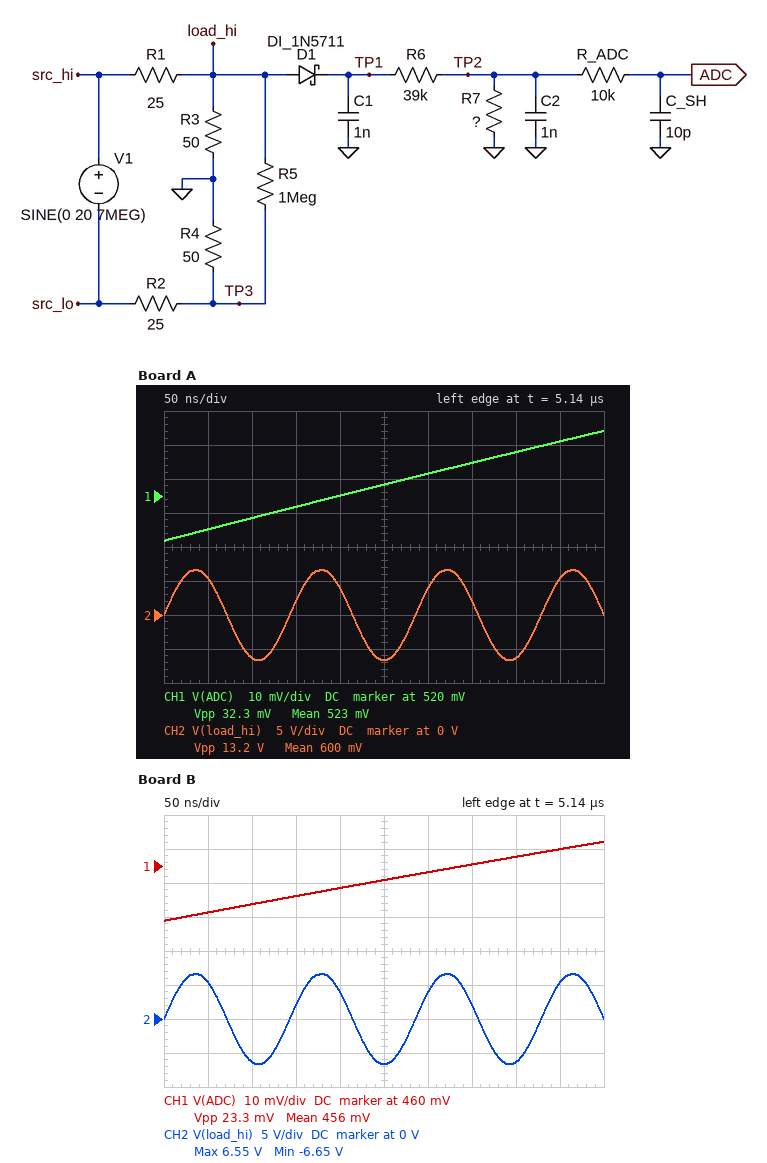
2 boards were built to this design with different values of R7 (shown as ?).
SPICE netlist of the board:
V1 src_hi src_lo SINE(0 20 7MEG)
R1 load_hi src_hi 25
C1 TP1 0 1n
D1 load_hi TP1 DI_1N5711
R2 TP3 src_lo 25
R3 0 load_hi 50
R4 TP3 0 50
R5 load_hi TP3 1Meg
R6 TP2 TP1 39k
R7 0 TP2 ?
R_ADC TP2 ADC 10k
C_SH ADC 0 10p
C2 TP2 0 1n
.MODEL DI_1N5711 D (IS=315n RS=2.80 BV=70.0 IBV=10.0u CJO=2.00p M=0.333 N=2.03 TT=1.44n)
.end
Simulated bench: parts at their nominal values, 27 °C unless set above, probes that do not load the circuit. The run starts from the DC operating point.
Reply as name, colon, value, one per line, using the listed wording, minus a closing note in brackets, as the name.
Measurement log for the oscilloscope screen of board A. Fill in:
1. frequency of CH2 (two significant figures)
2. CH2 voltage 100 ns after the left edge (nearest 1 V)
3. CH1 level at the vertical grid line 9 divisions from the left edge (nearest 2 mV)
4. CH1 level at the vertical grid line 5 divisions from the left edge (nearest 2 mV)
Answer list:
frequency of CH2: 7.0 MHz
CH2 voltage 100 ns after the left edge: -6 V
CH1 level at the vertical grid line 9 divisions from the left edge: 536 mV
CH1 level at the vertical grid line 5 divisions from the left edge: 524 mV
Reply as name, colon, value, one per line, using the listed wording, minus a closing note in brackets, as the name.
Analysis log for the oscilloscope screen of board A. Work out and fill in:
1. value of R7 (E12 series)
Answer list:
value of R7: 6.8 kΩ
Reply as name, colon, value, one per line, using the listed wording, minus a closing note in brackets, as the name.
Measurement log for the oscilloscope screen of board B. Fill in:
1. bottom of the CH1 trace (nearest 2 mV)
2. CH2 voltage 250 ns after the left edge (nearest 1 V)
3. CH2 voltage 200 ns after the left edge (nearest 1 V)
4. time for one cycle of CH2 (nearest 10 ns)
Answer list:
bottom of the CH1 trace: 444 mV
CH2 voltage 250 ns after the left edge: -7 V
CH2 voltage 200 ns after the left edge: 4 V
time for one cycle of CH2: 140 ns
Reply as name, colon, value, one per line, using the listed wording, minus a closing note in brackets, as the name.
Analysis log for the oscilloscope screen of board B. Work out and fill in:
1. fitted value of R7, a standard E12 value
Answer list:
fitted value of R7, a standard E12 value: 4.7 kΩ
